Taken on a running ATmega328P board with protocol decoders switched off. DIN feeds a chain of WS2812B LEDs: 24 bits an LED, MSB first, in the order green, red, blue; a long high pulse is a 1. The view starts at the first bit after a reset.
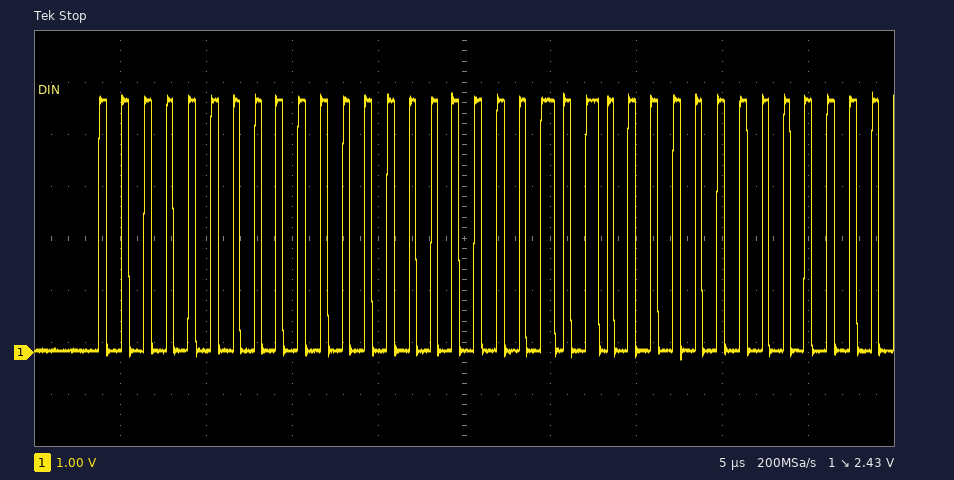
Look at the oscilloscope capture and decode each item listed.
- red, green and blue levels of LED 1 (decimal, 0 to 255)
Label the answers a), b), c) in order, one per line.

a) 0, 0, 10
